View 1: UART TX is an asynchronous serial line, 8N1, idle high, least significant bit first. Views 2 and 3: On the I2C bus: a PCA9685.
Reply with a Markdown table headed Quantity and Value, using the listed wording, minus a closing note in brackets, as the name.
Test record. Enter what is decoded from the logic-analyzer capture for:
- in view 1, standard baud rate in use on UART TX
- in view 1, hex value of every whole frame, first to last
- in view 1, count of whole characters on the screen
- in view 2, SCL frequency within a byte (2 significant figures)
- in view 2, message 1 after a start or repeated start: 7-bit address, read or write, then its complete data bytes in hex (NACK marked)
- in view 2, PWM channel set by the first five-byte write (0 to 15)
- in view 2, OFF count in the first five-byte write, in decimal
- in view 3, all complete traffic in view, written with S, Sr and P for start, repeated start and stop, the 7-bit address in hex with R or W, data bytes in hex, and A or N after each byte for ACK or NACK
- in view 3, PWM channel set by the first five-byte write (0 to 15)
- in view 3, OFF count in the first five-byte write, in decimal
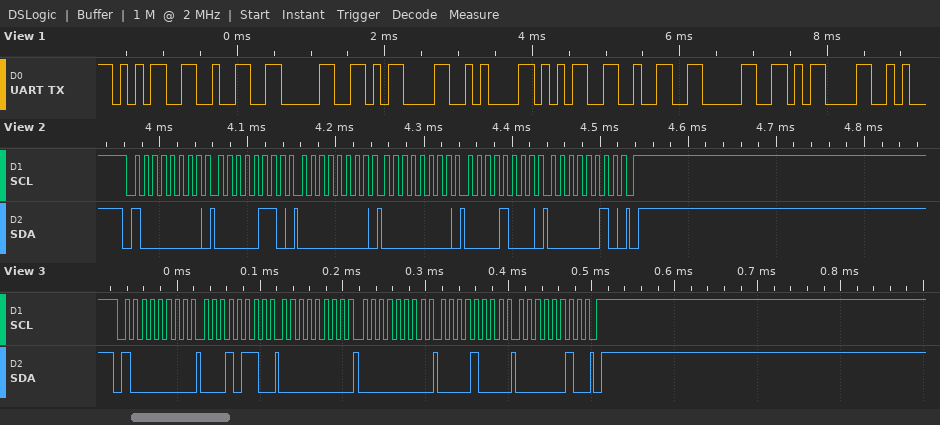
| Quantity | Value |
|---|---|
| in view 1, standard baud rate in use on UART TX | 9600 baud |
| in view 1, hex value of every whole frame, first to last | 35 32 30 0D 0A 35 32 30 0D |
| in view 1, count of whole characters on the screen | 9 |
| in view 2, SCL frequency within a byte | 100 kHz |
| in view 2, message 1 after a start or repeated start: 7-bit address, read or write, then its complete data bytes in hex | 0x40 write: 06 00 00 08 02 |
| in view 2, PWM channel set by the first five-byte write | 0 |
| in view 2, OFF count in the first five-byte write, in decimal | 520 |
| in view 3, all complete traffic in view, written with S, Sr and P for start, repeated start and stop, the 7-bit address in hex with R or W, data bytes in hex, and A or N after each byte for ACK or NACK | S 40W A 16 A 00 A 00 A 08 A 02 A P |
| in view 3, PWM channel set by the first five-byte write | 4 |
| in view 3, OFF count in the first five-byte write, in decimal | 520 |
